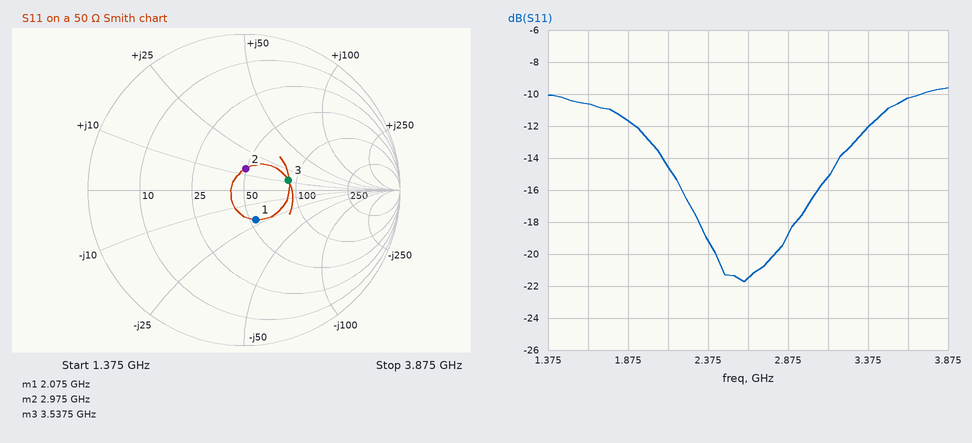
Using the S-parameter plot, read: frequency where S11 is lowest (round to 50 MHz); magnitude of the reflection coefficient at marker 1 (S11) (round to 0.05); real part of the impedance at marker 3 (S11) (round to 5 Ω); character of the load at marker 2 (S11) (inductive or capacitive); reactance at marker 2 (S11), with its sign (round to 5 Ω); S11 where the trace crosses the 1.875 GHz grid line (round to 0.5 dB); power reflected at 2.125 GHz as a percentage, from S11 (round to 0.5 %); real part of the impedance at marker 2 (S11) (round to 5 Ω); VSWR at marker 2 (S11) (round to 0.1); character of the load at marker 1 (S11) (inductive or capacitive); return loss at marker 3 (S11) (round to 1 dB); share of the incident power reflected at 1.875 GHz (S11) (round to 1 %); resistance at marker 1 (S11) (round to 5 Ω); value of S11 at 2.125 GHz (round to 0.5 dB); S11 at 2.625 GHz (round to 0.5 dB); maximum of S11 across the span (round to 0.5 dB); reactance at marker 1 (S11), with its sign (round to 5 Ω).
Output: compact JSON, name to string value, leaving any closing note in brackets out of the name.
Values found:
{"frequency where S11 is lowest": "2.60 GHz", "magnitude of the reflection coefficient at marker 1 (S11)": "0.20", "real part of the impedance at marker 3 (S11)": "90 Ω", "character of the load at marker 2 (S11)": "inductive", "reactance at marker 2 (S11), with its sign": "+15 Ω", "S11 where the trace crosses the 1.875 GHz grid line": "-11.5 dB", "power reflected at 2.125 GHz as a percentage, from S11": "3.5 %", "real part of the impedance at marker 2 (S11)": "50 Ω", "VSWR at marker 2 (S11)": "1.3", "character of the load at marker 1 (S11)": "capacitive", "return loss at marker 3 (S11)": "11 dB", "share of the incident power reflected at 1.875 GHz (S11)": "7 %", "resistance at marker 1 (S11)": "55 Ω", "value of S11 at 2.125 GHz": "-14.5 dB", "S11 at 2.625 GHz": "-21.5 dB", "maximum of S11 across the span": "-9.5 dB", "reactance at marker 1 (S11), with its sign": "-20 Ω"}
